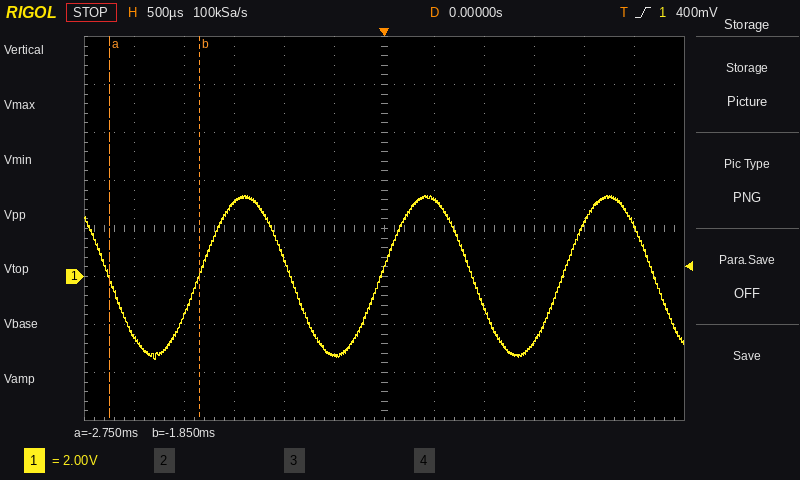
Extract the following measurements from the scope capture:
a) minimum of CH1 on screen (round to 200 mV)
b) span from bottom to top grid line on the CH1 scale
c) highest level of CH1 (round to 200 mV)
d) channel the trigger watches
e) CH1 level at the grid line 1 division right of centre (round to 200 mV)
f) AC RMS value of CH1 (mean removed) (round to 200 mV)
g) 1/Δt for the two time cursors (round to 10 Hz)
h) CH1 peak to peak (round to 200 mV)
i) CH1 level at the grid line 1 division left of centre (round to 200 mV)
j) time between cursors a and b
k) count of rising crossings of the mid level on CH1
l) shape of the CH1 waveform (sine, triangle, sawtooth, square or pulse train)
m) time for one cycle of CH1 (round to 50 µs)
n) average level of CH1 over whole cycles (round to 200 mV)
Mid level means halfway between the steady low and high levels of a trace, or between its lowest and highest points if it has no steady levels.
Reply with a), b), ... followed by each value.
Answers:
a) -3.4 V
b) 16 V
c) 3.4 V
d) CH1
e) 3.2 V
f) 2.4 V
g) 1.11 kHz
h) 6.8 V
i) -3.2 V
j) 900 µs
k) 3
l) sine
m) 1.80 ms
n) 0.0 V
